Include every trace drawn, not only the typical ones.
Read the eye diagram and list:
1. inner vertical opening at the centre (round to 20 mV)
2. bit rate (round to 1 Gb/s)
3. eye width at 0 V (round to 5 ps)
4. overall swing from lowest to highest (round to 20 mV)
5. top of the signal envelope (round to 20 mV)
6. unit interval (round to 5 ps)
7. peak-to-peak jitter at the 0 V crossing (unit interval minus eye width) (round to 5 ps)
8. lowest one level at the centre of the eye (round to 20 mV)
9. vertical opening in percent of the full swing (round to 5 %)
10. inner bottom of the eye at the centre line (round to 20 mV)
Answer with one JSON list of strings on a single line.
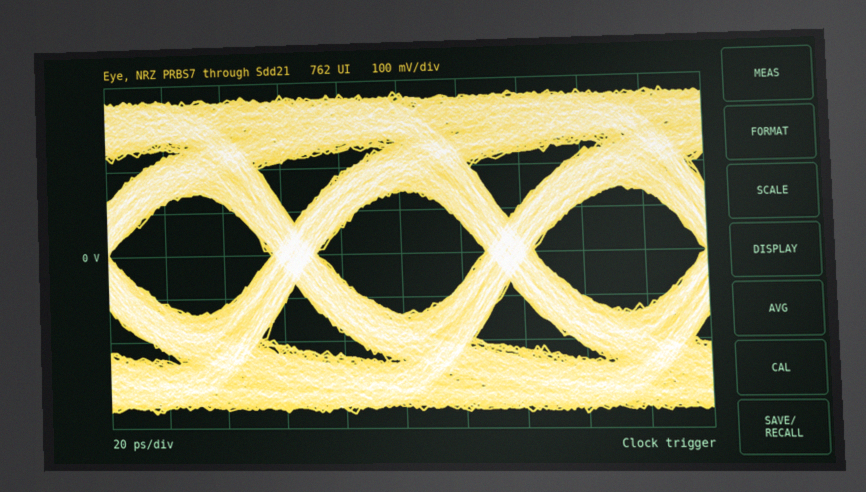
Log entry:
["280 mV", "14 Gb/s", "55 ps", "740 mV", "380 mV", "70 ps", "15 ps", "140 mV", "40 %", "-140 mV"]
